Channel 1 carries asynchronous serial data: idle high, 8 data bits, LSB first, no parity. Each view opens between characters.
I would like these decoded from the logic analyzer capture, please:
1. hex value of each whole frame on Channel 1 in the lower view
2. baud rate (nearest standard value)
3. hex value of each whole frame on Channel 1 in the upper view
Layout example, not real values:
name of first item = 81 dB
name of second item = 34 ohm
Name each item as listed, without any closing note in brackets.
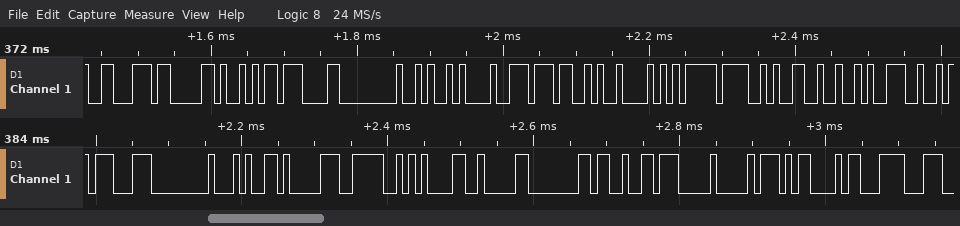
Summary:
hex value of each whole frame on Channel 1 in the lower view = C7, 00, 94, C1, 3E, 85, 82, 80, 93, 07, D0, 0D, E3
baud rate = 115200 baud
hex value of each whole frame on Channel 1 in the upper view = C6, 83, A9, 87, 00, 4A, C8, 37, 09, F5, 4F, 26, CA
